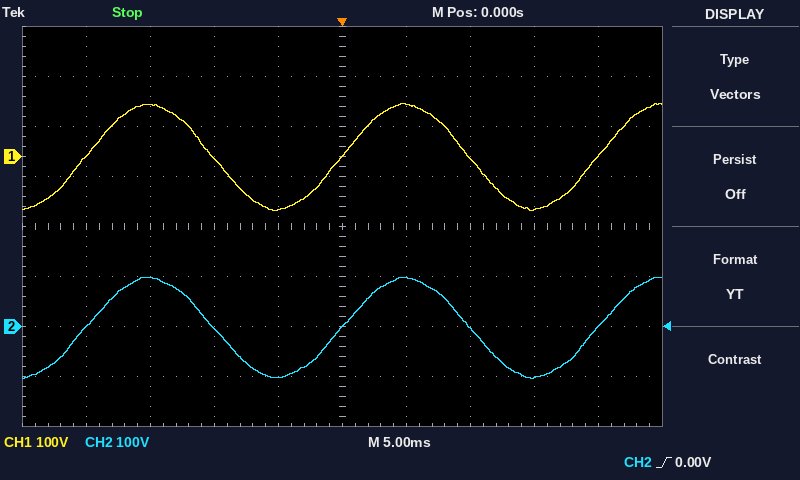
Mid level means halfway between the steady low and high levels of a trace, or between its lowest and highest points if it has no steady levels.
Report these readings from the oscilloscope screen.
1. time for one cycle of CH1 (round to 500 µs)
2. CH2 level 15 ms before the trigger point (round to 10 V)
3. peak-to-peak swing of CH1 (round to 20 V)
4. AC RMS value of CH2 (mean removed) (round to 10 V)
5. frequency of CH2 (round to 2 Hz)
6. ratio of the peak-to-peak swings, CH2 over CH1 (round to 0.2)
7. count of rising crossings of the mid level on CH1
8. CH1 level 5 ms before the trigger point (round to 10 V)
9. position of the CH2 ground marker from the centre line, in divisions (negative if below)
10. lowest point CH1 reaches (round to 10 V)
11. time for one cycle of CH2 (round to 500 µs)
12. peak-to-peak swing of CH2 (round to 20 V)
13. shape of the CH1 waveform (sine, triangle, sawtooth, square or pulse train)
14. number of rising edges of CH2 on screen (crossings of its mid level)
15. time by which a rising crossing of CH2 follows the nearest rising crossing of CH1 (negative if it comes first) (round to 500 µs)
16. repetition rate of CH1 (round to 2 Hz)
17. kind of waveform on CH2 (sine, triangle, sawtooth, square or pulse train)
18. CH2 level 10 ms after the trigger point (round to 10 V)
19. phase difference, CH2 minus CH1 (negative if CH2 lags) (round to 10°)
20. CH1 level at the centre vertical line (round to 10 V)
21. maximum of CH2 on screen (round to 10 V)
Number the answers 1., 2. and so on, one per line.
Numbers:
1. 20.0 ms
2. 100 V
3. 220 V
4. 70 V
5. 50 Hz
6. 1.0
7. 3
8. -110 V
9. -2.0 div
10. -110 V
11. 20.0 ms
12. 200 V
13. sine
14. 3
15. 0.0 ms
16. 50 Hz
17. sine
18. 0 V
19. 0°
20. 0 V
21. 100 V
